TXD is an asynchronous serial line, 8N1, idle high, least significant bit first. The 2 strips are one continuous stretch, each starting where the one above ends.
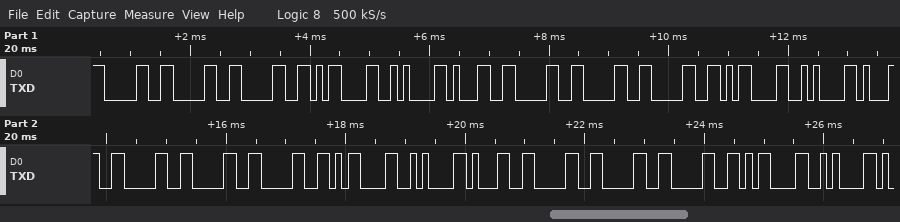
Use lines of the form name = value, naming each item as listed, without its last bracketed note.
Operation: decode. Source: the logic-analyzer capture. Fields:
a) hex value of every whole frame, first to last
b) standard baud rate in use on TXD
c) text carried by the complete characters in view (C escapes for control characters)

hex value of every whole frame, first to last = 0x30 0x30 0x30 0x0D 0x0A 0x31 0x30 0x30 0x30 0x0D 0x0A 0x31 0x30 0x30 0x30 0x0D 0x0A 0x31 0x30 0x30 0x30 0x0D 0x0A
standard baud rate in use on TXD = 9600 baud
text carried by the complete characters in view = "000\r\n1000\r\n1000\r\n1000\r\n"
